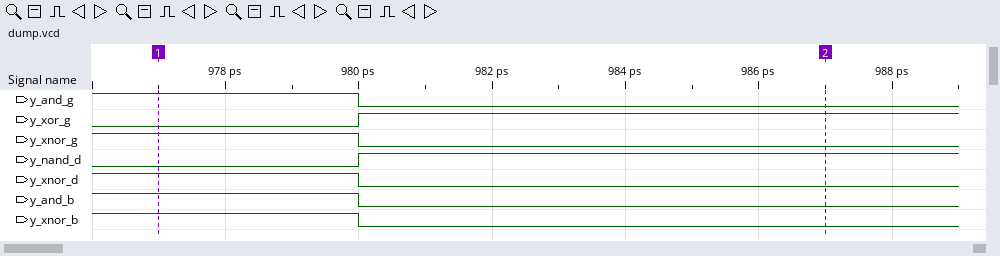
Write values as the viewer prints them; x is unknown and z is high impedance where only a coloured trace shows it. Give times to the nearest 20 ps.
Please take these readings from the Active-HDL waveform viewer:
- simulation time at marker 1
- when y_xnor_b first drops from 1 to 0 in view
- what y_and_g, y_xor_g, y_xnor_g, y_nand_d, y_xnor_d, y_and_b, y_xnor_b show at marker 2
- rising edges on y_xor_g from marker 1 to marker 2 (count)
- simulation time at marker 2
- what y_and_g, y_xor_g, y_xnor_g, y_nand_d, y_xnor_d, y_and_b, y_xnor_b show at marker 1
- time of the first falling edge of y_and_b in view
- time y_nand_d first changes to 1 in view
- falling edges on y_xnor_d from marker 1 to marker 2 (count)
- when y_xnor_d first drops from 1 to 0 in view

980 ps
980 ps
y_and_g=0, y_xor_g=1, y_xnor_g=0, y_nand_d=1, y_xnor_d=0, y_and_b=0, y_xnor_b=0
1
980 ps
y_and_g=1, y_xor_g=0, y_xnor_g=1, y_nand_d=0, y_xnor_d=1, y_and_b=1, y_xnor_b=1
980 ps
980 ps
1
980 ps
